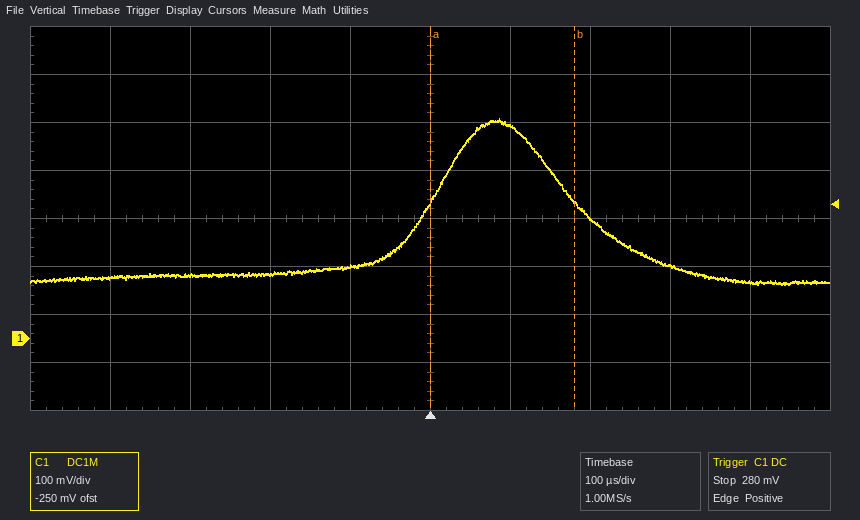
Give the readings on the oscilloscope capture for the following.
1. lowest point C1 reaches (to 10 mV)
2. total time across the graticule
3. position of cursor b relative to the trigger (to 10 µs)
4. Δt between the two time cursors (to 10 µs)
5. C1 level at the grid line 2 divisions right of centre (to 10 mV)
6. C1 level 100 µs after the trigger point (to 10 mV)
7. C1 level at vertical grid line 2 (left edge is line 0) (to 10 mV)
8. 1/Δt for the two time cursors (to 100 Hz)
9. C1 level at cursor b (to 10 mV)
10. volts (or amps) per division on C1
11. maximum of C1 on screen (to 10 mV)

110 mV
1 ms
+180 µs
180 µs
250 mV
440 mV
130 mV
5.6 kHz
280 mV
100 mV
460 mV
